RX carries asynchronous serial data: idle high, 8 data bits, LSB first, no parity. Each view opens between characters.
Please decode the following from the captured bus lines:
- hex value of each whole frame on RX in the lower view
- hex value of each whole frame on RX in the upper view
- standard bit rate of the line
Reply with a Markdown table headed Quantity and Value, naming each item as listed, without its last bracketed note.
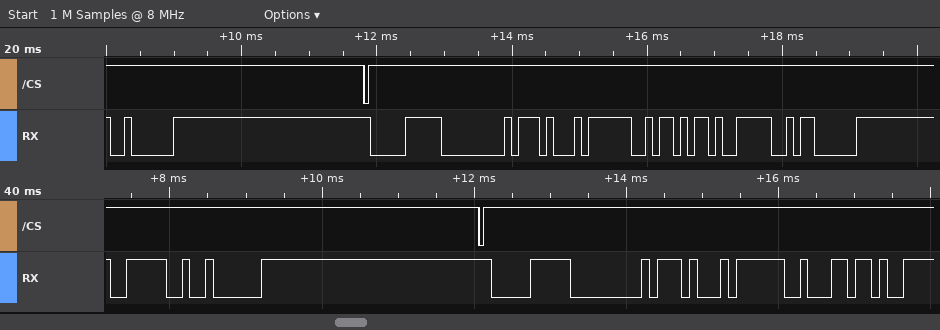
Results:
| Quantity | Value |
|---|---|
| hex value of each whole frame on RX in the lower view | 3E, 02, F0, 00, 17, 3F, 6C |
| hex value of each whole frame on RX in the upper view | 02, F0, 00, 17, 3F, 6B, 3E, 03 |
| standard bit rate of the line | 9600 baud |
